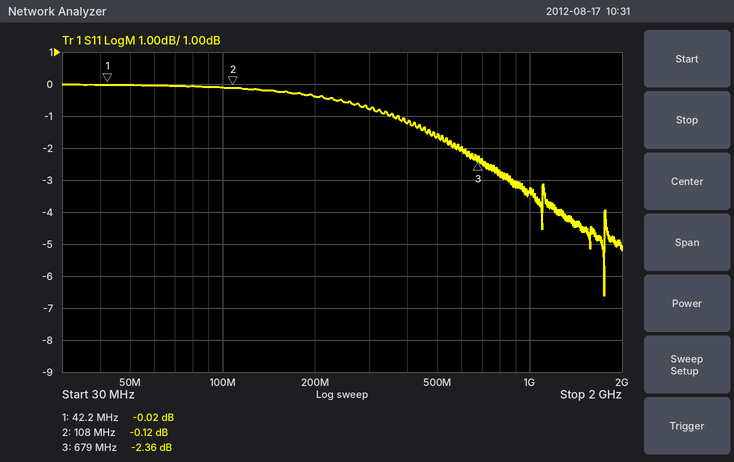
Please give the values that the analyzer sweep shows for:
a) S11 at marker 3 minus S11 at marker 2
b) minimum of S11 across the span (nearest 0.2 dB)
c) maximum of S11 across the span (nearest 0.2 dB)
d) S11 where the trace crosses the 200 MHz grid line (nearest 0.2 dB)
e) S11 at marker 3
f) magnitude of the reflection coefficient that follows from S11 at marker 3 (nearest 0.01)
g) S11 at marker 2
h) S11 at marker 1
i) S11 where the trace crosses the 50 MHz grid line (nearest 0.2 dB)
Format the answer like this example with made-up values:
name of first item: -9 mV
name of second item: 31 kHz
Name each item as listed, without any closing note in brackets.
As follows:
S11 at marker 3 minus S11 at marker 2: -2.24 dB
minimum of S11 across the span: -6.6 dB
maximum of S11 across the span: 0.0 dB
S11 where the trace crosses the 200 MHz grid line: -0.4 dB
S11 at marker 3: -2.36 dB
magnitude of the reflection coefficient that follows from S11 at marker 3: 0.76
S11 at marker 2: -0.12 dB
S11 at marker 1: -0.02 dB
S11 where the trace crosses the 50 MHz grid line: 0.0 dB
